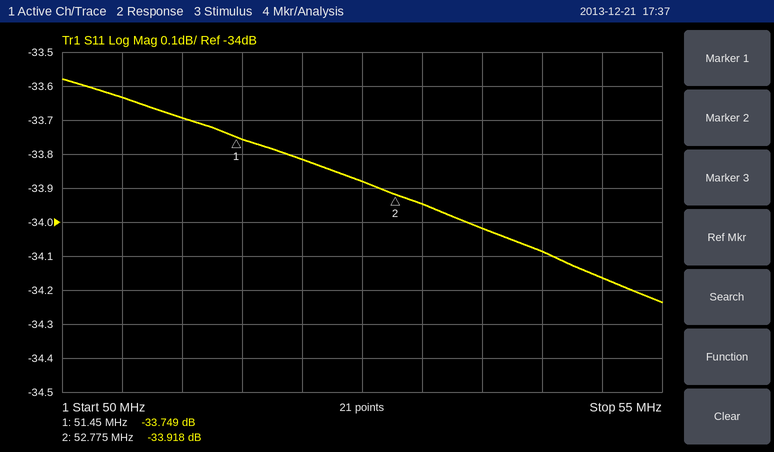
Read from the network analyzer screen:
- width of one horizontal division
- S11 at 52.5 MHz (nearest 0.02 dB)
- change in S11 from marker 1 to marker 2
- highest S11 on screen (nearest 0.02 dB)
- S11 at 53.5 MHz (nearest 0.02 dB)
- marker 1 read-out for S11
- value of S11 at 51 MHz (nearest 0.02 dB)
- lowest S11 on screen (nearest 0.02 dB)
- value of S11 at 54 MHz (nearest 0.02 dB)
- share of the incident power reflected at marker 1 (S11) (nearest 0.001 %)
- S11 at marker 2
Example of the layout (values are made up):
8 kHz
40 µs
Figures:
500 kHz
-33.88 dB
-0.169 dB
-33.58 dB
-34.02 dB
-33.749 dB
-33.70 dB
-34.24 dB
-34.08 dB
0.042 %
-33.918 dB
